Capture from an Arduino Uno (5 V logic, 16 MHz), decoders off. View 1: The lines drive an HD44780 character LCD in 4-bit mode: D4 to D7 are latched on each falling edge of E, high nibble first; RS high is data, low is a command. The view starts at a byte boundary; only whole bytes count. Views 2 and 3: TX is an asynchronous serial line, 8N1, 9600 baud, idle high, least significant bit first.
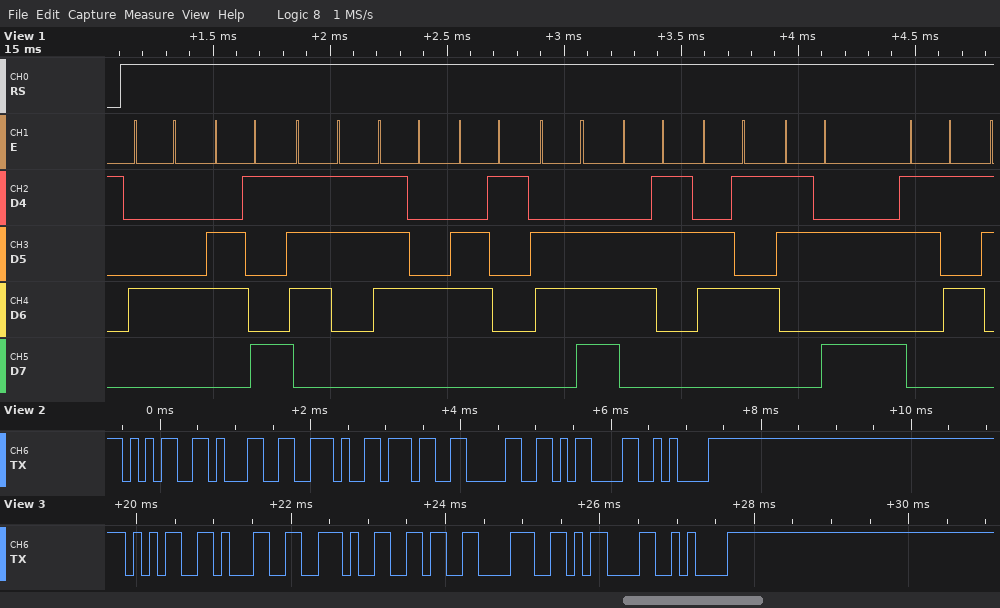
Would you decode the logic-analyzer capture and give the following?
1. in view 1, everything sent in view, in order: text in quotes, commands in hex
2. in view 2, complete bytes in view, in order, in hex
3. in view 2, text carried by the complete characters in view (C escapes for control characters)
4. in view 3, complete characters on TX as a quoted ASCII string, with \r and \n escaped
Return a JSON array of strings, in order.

["\"Distance:5\"", "35 31 2E 37 30 0D 0A", "\"51.70\\r\\n\"", "\"51.68\\r\\n\""]
